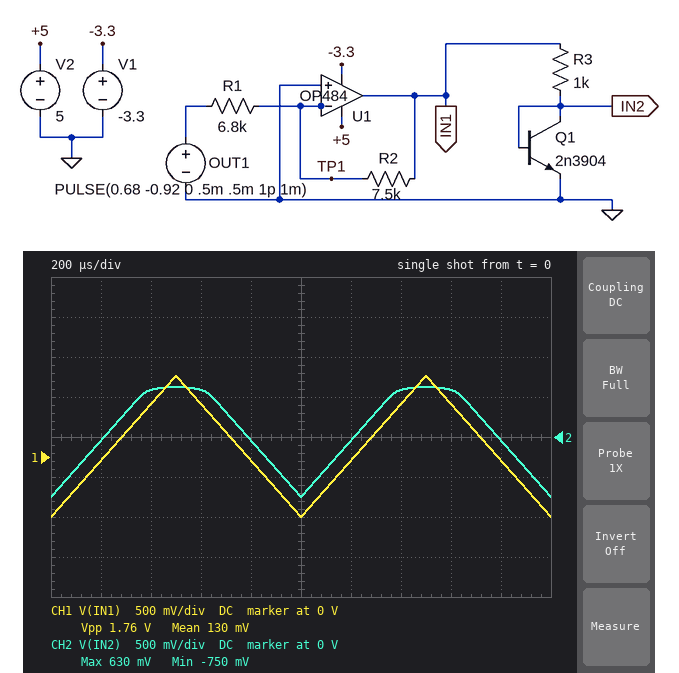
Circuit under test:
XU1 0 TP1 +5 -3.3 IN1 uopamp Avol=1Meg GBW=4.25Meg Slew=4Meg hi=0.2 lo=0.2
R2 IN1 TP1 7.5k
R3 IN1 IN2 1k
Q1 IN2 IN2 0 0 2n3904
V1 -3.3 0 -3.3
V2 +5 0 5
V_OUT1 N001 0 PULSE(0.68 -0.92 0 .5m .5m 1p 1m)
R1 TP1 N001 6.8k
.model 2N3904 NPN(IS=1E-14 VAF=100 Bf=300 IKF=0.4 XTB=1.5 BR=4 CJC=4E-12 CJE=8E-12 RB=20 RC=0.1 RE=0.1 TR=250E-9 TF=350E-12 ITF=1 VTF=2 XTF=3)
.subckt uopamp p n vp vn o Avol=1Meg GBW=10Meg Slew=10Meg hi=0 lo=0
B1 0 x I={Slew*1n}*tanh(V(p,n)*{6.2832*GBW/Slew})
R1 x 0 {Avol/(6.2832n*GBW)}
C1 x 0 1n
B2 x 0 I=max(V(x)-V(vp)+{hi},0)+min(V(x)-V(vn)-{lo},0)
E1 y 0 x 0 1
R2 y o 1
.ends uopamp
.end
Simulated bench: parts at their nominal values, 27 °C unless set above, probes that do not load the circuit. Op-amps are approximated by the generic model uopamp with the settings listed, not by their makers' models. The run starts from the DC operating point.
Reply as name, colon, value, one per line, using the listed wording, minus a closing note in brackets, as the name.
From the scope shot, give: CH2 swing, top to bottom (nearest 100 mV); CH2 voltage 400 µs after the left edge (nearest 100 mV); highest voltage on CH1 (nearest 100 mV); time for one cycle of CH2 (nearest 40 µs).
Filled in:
CH2 swing, top to bottom: 1.4 V
CH2 voltage 400 µs after the left edge: 600 mV
highest voltage on CH1: 1.0 V
time for one cycle of CH2: 1.00 ms
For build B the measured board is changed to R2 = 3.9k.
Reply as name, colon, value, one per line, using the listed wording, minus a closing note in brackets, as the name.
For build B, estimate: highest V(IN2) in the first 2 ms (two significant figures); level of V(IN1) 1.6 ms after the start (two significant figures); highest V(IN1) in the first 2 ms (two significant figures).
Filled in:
highest V(IN2) in the first 2 ms: 520 mV
level of V(IN1) 1.6 ms after the start: 340 mV
highest V(IN1) in the first 2 ms: 530 mV
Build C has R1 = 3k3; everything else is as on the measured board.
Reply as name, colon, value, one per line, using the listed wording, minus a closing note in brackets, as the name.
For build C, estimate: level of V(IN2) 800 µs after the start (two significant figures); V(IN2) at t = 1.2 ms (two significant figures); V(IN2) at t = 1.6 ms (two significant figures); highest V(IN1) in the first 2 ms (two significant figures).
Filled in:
level of V(IN2) 800 µs after the start: -90 mV
V(IN2) at t = 1.2 ms: -92 mV
V(IN2) at t = 1.6 ms: 650 mV
highest V(IN1) in the first 2 ms: 2.1 V
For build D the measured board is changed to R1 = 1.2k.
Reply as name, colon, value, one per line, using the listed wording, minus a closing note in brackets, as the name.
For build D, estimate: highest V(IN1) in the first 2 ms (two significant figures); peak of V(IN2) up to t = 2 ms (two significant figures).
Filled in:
highest V(IN1) in the first 2 ms: 4.8 V
peak of V(IN2) up to t = 2 ms: 690 mV
